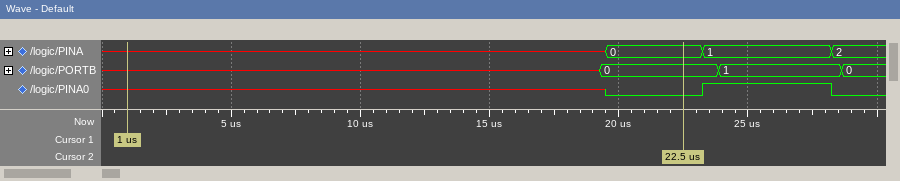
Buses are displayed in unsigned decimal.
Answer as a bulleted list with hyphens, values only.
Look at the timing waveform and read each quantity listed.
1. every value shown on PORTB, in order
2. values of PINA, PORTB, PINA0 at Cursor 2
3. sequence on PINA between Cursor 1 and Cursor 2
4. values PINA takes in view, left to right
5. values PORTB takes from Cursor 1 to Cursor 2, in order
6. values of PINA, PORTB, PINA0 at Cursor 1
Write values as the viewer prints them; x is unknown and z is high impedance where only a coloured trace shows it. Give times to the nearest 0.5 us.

- x, 0, 1, 0
- PINA=0, PORTB=0, PINA0=0
- x, 0
- x, 0, 1, 2
- x, 0
- PINA=x, PORTB=x, PINA0=x
